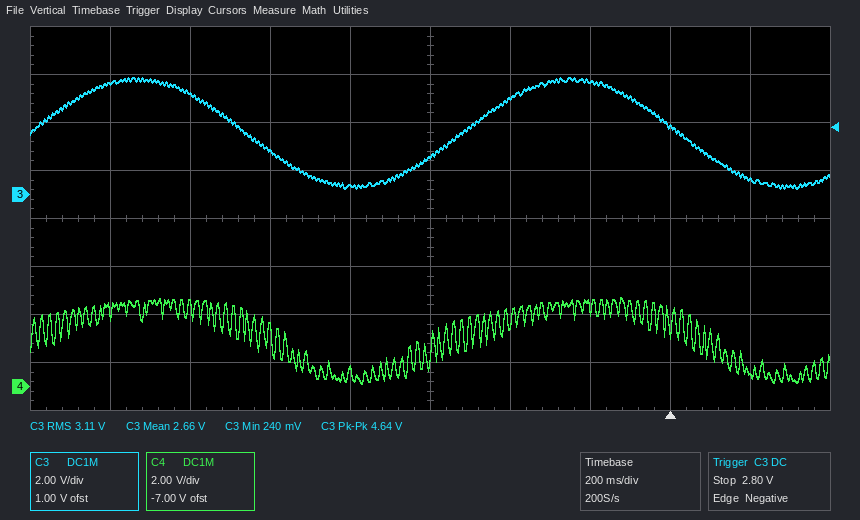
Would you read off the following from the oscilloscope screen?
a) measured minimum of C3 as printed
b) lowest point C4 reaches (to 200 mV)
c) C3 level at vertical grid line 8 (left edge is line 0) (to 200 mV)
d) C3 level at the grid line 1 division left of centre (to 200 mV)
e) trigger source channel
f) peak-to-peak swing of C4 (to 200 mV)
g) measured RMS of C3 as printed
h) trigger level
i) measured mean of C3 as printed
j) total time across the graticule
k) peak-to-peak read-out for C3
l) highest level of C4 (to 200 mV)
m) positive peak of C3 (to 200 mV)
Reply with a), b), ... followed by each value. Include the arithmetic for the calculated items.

a) 240 mV
b) 200 mV
c) 2.8 V
d) 400 mV
e) C3
f) 3.8 V − (200 mV) = 3.6 V
g) 3.11 V
h) 2.80 V
i) 2.66 V
j) 2 s
k) 4.64 V
l) 3.8 V
m) 4.8 V
